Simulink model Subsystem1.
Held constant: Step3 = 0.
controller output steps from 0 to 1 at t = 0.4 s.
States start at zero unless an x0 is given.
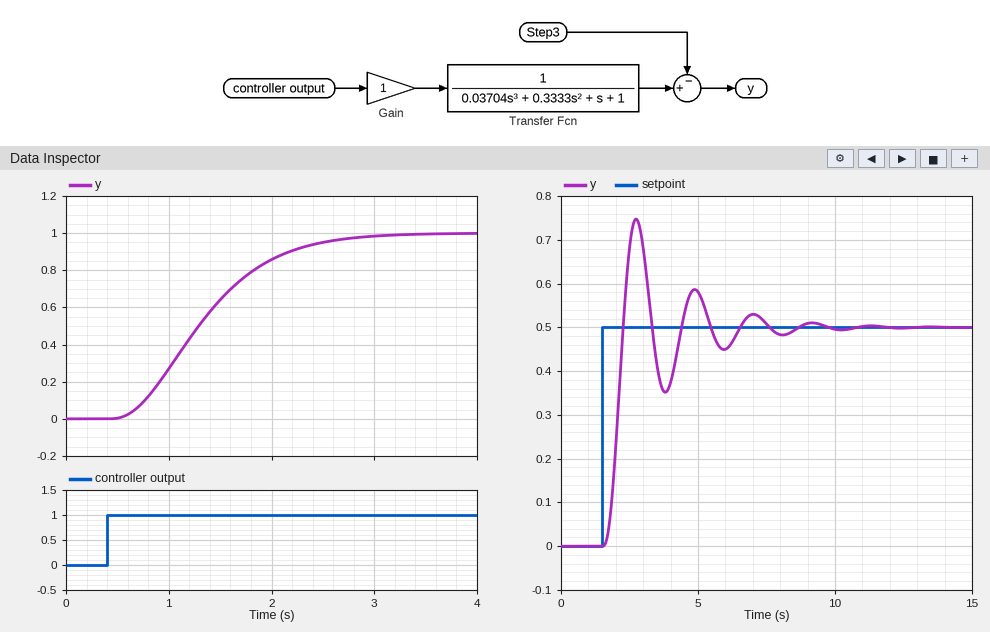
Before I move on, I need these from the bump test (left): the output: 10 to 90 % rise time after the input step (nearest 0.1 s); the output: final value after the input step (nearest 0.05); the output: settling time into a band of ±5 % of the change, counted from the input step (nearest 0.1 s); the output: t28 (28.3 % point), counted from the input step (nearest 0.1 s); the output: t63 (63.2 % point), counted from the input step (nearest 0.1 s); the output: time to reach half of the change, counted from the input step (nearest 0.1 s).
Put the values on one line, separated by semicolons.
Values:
1.4 s; 1.00; 2.1 s; 0.6 s; 1.1 s; 0.9 s
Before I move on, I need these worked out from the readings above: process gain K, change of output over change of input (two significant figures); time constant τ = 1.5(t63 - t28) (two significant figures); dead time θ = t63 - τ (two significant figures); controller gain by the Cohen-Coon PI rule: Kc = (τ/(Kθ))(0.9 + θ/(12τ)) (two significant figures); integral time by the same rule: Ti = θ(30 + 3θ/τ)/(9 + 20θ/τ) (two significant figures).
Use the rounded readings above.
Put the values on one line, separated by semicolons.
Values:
1.0; 0.75 s; 0.35 s; 2.0; 0.60 s
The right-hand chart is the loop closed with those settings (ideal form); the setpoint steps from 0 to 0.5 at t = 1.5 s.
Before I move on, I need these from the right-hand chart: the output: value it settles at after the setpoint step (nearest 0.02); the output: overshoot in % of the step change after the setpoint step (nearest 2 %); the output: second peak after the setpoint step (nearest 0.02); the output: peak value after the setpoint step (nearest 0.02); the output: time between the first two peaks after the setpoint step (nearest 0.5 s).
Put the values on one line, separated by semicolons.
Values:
0.50; 50 %; 0.58; 0.74; 2.0 s
